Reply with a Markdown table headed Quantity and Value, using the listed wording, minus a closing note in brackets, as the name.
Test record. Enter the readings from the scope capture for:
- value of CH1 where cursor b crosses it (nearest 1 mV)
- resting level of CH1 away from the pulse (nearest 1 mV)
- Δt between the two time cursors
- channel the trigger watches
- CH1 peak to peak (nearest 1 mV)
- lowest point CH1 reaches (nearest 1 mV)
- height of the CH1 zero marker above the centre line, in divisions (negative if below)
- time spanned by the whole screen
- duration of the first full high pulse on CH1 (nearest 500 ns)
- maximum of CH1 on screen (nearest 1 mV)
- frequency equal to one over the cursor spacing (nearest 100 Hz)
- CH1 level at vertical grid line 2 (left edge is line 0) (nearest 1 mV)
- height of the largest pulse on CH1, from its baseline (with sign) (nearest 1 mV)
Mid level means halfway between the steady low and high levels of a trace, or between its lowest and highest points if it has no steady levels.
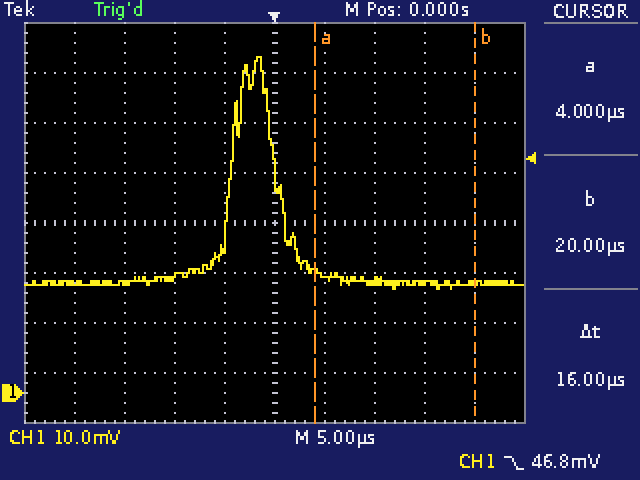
| Quantity | Value |
|---|---|
| value of CH1 where cursor b crosses it | 22 mV |
| resting level of CH1 away from the pulse | 22 mV |
| Δt between the two time cursors | 16 µs |
| channel the trigger watches | CH1 |
| CH1 peak to peak | 46 mV |
| lowest point CH1 reaches | 21 mV |
| height of the CH1 zero marker above the centre line, in divisions | -3.4 div |
| time spanned by the whole screen | 50 µs |
| duration of the first full high pulse on CH1 | 4.5 µs |
| maximum of CH1 on screen | 67 mV |
| frequency equal to one over the cursor spacing | 62.5 kHz |
| CH1 level at vertical grid line 2 (left edge is line 0) | 22 mV |
| height of the largest pulse on CH1, from its baseline (with sign) | +45 mV |
